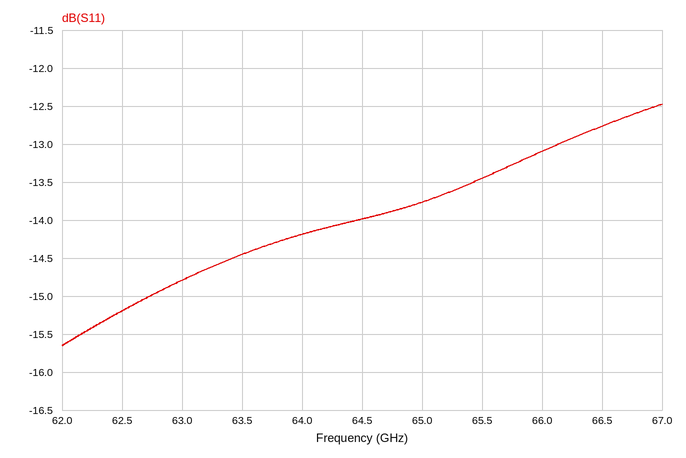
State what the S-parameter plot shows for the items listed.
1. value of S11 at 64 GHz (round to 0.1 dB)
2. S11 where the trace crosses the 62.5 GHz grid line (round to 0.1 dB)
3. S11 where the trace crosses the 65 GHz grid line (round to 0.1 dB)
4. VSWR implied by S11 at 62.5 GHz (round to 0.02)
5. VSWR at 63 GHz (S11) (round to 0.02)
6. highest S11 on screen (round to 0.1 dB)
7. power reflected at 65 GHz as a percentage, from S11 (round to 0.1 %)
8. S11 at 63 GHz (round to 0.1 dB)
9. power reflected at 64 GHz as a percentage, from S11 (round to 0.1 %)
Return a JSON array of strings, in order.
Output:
["-14.2 dB", "-15.2 dB", "-13.8 dB", "1.42", "1.44", "-12.5 dB", "4.2 %", "-14.8 dB", "3.8 %"]
